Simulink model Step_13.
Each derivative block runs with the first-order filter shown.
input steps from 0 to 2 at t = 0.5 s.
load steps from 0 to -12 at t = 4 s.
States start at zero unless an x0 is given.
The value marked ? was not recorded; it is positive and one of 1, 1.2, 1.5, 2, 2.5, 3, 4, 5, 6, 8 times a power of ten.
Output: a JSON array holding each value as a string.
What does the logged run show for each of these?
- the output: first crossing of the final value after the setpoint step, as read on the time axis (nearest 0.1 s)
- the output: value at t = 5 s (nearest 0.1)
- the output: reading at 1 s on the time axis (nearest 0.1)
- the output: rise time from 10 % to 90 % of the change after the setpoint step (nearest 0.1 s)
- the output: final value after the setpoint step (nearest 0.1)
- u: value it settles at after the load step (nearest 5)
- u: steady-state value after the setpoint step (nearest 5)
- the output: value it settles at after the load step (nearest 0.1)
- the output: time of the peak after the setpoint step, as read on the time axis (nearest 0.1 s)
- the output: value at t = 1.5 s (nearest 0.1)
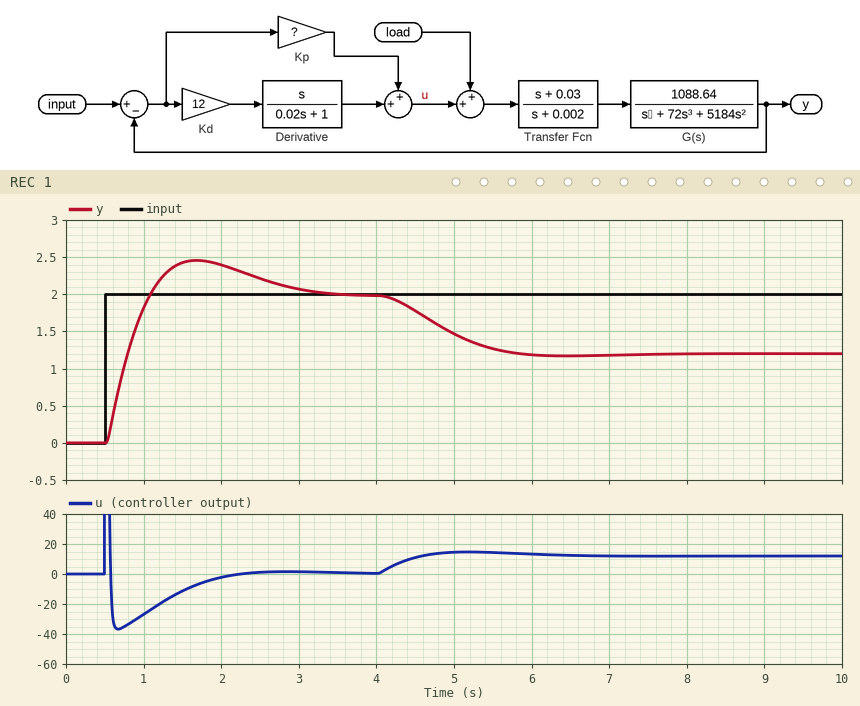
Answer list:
["1.1 s", "1.5", "1.8", "0.4 s", "2.0", "10", "0", "1.2", "1.7 s", "2.4"]
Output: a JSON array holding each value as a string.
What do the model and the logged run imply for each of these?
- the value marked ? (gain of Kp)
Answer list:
["15"]
